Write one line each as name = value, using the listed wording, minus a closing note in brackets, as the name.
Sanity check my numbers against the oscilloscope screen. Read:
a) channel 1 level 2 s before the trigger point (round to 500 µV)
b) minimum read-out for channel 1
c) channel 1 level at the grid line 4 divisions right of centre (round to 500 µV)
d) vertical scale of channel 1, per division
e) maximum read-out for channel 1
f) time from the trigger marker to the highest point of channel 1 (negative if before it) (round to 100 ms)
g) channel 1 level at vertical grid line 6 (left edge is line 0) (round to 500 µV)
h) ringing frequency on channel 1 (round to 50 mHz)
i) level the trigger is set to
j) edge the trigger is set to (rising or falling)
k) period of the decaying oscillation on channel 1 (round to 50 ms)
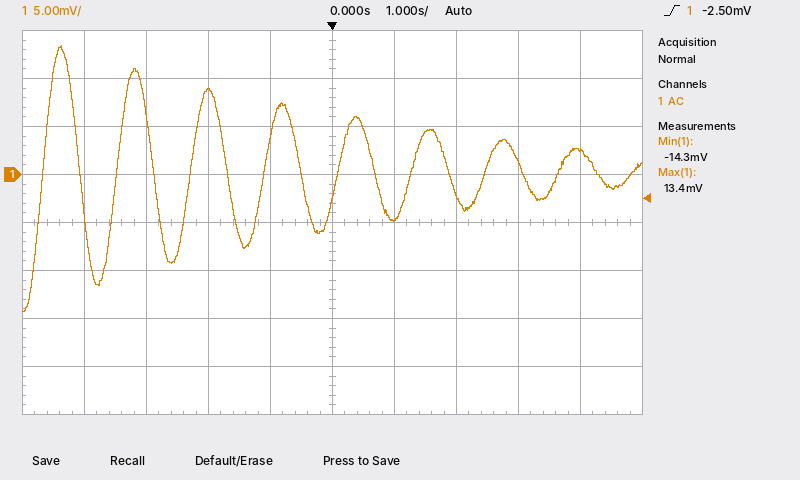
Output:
channel 1 level 2 s before the trigger point = 9.0 mV
minimum read-out for channel 1 = -14.3 mV
channel 1 level at the grid line 4 divisions right of centre = 2.5 mV
vertical scale of channel 1, per division = 5 mV
maximum read-out for channel 1 = 13.4 mV
time from the trigger marker to the highest point of channel 1 (negative if before it) = -4.4 s
channel 1 level at vertical grid line 6 (left edge is line 0) = -4.5 mV
ringing frequency on channel 1 = 850 mHz
level the trigger is set to = -2.50 mV
edge the trigger is set to = rising
period of the decaying oscillation on channel 1 = 1.20 s
